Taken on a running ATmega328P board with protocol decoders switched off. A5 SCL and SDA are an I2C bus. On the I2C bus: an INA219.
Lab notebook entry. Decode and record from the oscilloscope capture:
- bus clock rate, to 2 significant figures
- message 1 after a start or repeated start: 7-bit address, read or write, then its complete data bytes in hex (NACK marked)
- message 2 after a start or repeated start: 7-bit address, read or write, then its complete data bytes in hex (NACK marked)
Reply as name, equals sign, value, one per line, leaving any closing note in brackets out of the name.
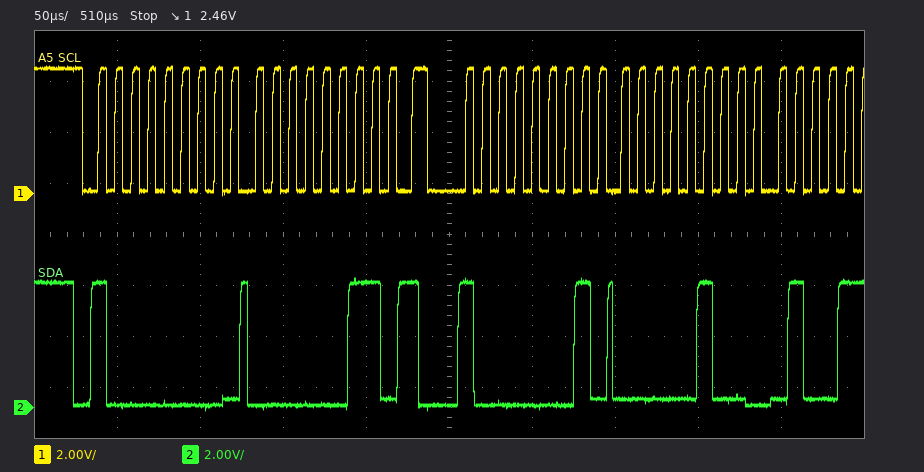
bus clock rate, to 2 significant figures = 100 kHz
message 1 after a start or repeated start: 7-bit address, read or write, then its complete data bytes in hex = 0x40 write: 03
message 2 after a start or repeated start: 7-bit address, read or write, then its complete data bytes in hex = 0x40 read: 04
